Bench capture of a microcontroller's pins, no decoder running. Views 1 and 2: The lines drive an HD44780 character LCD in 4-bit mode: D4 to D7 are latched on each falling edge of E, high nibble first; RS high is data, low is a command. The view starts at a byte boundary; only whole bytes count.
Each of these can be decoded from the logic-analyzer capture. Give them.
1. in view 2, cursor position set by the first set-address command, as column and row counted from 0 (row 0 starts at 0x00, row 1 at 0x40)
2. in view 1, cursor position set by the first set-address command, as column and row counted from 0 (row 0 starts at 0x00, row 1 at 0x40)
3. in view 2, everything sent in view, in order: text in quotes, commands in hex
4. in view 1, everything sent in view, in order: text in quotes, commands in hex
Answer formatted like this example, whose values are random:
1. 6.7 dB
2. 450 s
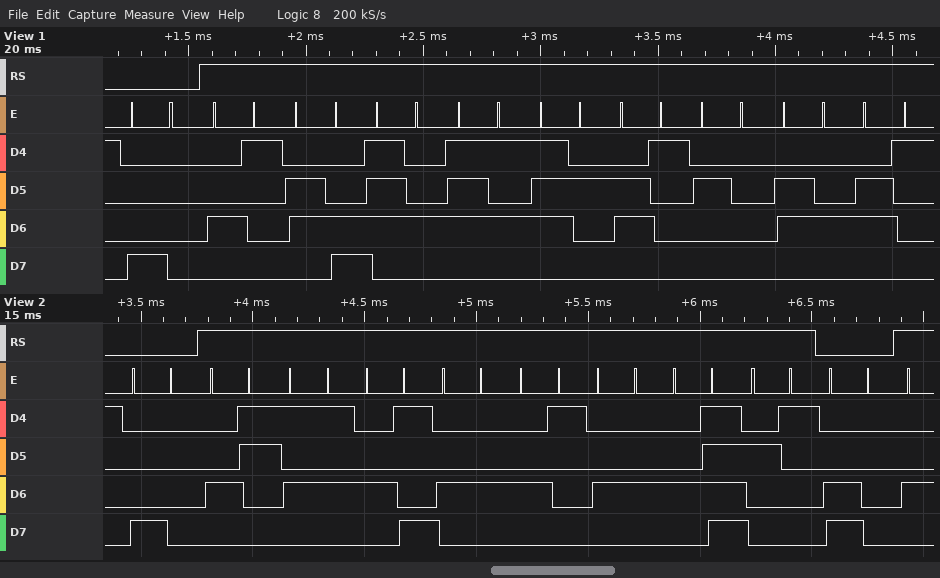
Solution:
1. column 0, row 0
2. column 0, row 0
3. 0x80 "CUIDADO!" 0xC0
4. 0x80 "Altura da"
